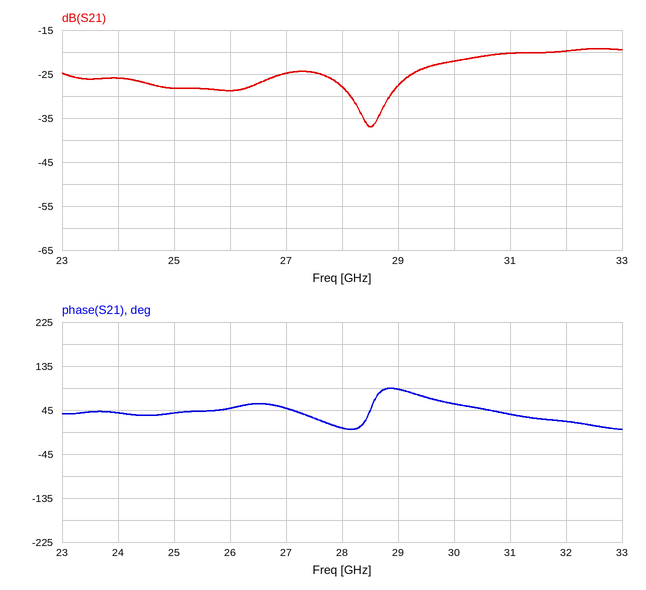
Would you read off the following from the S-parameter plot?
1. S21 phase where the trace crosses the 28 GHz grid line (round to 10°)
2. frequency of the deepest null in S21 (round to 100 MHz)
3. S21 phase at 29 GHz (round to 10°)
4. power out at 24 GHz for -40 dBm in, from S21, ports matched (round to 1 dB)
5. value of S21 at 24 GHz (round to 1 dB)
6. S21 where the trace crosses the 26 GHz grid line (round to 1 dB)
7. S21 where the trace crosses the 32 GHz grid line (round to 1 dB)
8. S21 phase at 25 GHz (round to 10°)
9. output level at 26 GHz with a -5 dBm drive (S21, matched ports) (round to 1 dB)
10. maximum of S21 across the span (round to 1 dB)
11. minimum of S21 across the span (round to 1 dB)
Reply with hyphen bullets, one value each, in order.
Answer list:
- 10°
- 28.5 GHz
- 90°
- -66 dBm
- -26 dB
- -29 dB
- -20 dB
- 40°
- -34 dBm
- -19 dB
- -37 dB
